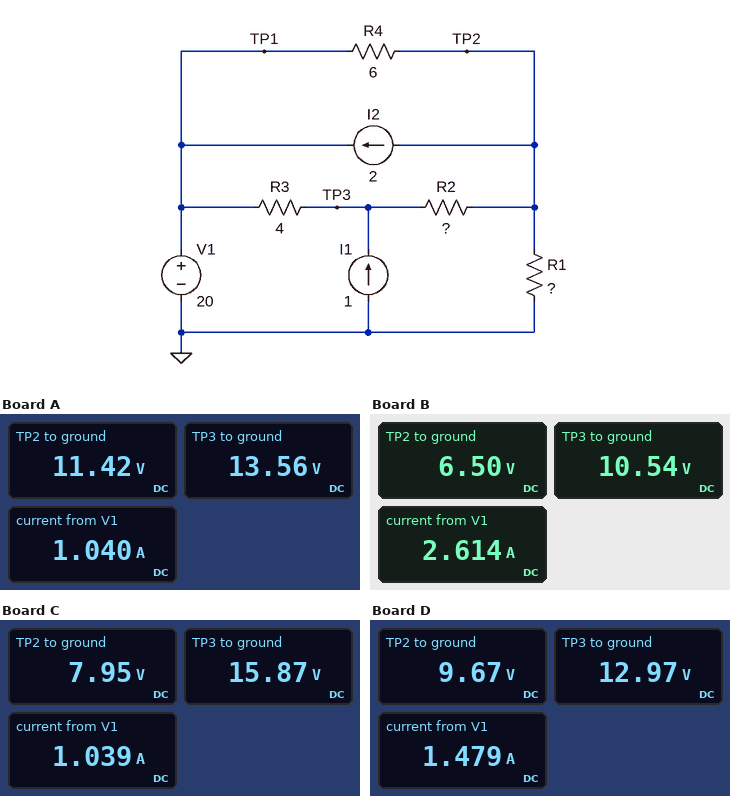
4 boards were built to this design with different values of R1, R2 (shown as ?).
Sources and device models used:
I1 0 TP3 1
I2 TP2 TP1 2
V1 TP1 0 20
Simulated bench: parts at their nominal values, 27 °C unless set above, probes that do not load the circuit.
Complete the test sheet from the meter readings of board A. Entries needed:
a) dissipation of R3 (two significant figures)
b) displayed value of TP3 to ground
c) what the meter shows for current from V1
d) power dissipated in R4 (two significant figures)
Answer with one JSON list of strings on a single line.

["10 W", "13.56 V", "1.040 A", "12 W"]
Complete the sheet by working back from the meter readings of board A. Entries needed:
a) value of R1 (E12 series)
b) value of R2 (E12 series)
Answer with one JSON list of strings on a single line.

["5.6 Ω", "0.82 Ω"]
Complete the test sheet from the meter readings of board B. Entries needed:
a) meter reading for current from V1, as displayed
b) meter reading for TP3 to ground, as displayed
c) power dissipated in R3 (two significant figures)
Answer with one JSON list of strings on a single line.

["2.614 A", "10.54 V", "22 W"]
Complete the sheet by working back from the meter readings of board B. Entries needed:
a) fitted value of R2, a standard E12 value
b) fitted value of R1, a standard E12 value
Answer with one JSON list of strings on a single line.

["1.2 Ω", "1.8 Ω"]
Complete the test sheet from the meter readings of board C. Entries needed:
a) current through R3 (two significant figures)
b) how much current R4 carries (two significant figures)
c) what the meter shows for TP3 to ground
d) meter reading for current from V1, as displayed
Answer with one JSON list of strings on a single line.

["1.0 A", "2.0 A", "15.87 V", "1.039 A"]
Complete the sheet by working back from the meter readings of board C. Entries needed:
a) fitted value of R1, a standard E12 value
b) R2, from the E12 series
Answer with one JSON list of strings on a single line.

["3.9 Ω", "3.9 Ω"]
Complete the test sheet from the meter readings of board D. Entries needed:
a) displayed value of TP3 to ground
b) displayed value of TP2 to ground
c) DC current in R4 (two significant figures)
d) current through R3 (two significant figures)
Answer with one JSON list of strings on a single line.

["12.97 V", "9.67 V", "1.7 A", "1.8 A"]
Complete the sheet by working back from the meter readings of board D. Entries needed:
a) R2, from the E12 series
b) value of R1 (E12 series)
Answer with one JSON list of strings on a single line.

["1.2 Ω", "3.9 Ω"]
